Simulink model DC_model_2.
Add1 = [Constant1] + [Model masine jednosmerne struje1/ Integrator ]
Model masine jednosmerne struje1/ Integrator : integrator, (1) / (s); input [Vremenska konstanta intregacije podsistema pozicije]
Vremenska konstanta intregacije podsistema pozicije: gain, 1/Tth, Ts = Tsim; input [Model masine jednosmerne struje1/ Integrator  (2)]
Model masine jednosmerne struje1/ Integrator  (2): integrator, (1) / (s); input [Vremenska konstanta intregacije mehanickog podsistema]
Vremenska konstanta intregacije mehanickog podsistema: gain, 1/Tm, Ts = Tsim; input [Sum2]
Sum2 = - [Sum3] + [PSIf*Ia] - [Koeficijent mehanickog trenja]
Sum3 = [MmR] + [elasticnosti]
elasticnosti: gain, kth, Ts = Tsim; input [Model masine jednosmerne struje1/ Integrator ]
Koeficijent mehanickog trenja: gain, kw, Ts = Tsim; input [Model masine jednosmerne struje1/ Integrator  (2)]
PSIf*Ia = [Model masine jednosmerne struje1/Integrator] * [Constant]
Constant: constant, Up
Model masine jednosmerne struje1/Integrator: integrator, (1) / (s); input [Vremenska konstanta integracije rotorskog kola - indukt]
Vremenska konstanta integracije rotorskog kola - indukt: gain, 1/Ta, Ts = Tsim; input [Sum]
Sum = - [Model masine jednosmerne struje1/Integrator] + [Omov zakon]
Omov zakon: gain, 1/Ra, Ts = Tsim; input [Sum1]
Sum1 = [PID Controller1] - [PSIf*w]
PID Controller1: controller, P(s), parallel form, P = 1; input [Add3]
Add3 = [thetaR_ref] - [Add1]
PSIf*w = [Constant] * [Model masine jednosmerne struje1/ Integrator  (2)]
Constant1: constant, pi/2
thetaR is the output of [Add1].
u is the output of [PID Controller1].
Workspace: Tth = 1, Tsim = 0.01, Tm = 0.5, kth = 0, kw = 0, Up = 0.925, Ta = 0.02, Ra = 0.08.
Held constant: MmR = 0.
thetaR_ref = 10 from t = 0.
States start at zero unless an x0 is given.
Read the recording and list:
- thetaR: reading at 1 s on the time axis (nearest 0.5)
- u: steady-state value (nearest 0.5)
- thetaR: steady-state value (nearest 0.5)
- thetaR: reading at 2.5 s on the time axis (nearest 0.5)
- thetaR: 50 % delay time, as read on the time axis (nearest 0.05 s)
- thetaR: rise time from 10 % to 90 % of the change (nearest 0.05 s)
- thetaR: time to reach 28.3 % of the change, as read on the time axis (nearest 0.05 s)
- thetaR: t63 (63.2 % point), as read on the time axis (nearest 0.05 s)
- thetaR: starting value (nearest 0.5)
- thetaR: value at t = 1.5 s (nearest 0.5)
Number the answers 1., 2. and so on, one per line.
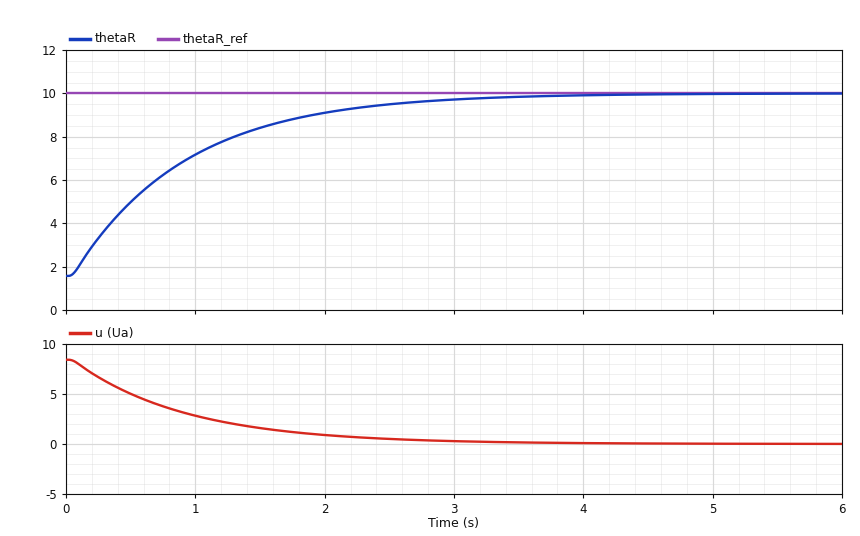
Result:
1. 7.0
2. 0.0
3. 10.0
4. 9.5
5. 0.65 s
6. 1.90 s
7. 0.35 s
8. 0.90 s
9. 1.5
10. 8.5
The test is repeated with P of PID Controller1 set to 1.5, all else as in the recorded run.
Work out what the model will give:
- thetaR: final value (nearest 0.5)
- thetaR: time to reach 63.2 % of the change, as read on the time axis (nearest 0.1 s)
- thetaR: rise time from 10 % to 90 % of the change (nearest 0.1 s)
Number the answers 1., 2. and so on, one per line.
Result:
1. 10.0
2. 0.6 s
3. 1.2 s
